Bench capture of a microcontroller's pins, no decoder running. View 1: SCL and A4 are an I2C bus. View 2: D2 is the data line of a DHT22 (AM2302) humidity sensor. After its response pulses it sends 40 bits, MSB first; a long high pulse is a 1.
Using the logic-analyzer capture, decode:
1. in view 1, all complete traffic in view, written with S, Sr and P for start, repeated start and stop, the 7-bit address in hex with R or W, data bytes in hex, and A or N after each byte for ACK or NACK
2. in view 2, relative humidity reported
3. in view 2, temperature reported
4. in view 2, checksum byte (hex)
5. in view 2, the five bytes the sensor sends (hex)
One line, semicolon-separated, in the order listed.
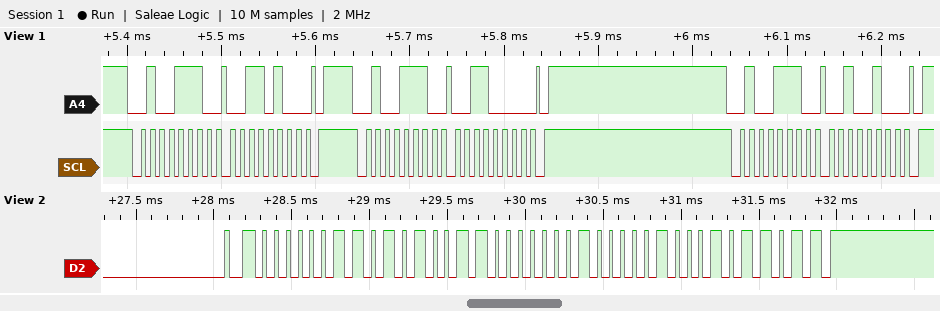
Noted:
S 27W A 34 A P S 27W A 30 A P S 27W A 24 A P; 85.1 %; 26.0 °C; 0x5B; 03 53 01 04 5B
